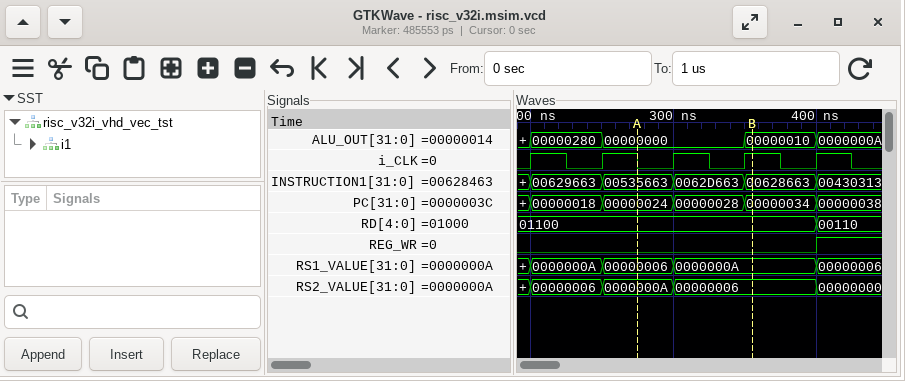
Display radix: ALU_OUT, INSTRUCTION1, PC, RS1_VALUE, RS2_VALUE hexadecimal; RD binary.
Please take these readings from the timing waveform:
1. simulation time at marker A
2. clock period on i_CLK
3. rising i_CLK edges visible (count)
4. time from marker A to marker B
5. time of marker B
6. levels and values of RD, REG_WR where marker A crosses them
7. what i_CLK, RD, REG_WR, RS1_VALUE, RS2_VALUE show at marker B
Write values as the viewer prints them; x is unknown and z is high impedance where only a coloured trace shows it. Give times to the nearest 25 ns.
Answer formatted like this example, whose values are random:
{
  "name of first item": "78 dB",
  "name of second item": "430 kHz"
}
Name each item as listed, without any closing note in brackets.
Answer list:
{
  "simulation time at marker A": "275 ns",
  "clock period on i_CLK": "50 ns",
  "rising i_CLK edges visible": "5",
  "time from marker A to marker B": "75 ns",
  "time of marker B": "350 ns",
  "levels and values of RD, REG_WR where marker A crosses them": "RD=01100, REG_WR=0",
  "what i_CLK, RD, REG_WR, RS1_VALUE, RS2_VALUE show at marker B": "i_CLK=1, RD=01100, REG_WR=0, RS1_VALUE=0000000A, RS2_VALUE=00000006"
}
